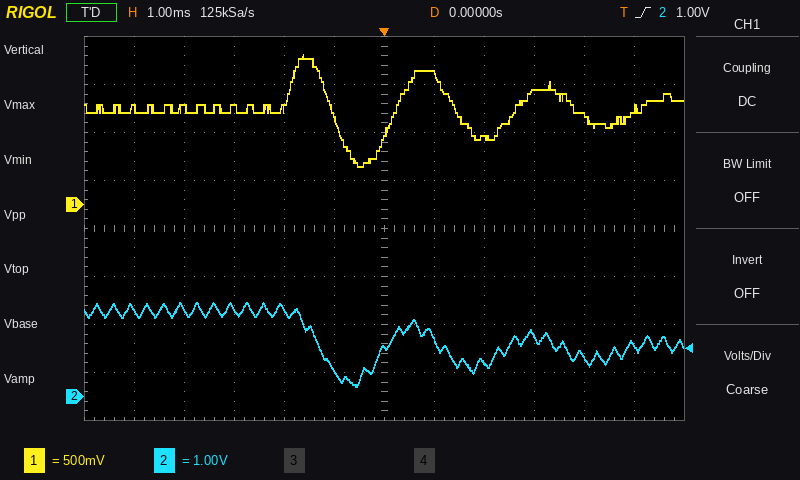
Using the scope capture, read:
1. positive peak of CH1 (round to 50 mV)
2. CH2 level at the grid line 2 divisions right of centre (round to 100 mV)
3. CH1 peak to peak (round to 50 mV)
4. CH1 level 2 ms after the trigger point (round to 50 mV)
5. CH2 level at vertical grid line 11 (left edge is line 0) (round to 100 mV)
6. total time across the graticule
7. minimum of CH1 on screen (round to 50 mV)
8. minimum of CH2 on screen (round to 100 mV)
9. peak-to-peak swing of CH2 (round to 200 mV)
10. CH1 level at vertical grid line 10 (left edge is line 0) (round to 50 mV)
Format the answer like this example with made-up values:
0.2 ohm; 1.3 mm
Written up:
1.55 V; 700 mV; 1.15 V; 700 mV; 1.1 V; 12 ms; 400 mV; 200 mV; 1.8 V; 950 mV
